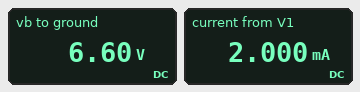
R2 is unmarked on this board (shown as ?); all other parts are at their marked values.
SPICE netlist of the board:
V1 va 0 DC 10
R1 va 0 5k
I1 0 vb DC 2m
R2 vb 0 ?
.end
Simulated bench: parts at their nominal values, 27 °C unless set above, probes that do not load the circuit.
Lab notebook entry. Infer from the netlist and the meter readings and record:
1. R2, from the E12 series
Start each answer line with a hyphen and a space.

- 3.3 kΩ
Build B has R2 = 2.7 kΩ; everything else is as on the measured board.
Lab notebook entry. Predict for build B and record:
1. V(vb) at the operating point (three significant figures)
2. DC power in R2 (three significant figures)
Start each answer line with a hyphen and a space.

- 5.40 V
- 10.8 mW
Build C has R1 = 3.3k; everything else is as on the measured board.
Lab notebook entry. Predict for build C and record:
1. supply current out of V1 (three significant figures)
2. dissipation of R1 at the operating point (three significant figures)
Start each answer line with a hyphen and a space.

- 3.03 mA
- 30.3 mW
